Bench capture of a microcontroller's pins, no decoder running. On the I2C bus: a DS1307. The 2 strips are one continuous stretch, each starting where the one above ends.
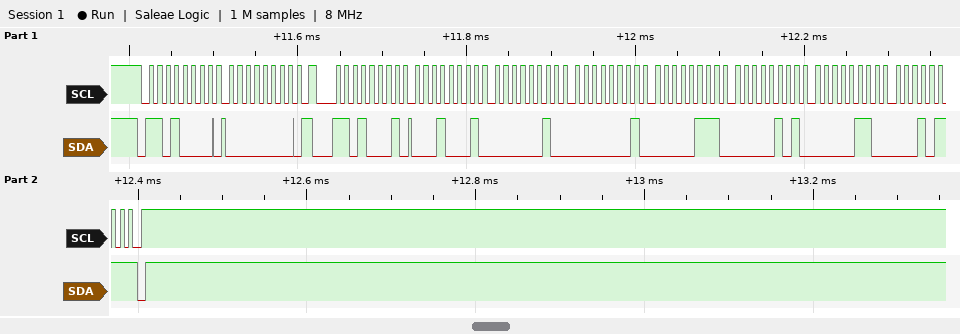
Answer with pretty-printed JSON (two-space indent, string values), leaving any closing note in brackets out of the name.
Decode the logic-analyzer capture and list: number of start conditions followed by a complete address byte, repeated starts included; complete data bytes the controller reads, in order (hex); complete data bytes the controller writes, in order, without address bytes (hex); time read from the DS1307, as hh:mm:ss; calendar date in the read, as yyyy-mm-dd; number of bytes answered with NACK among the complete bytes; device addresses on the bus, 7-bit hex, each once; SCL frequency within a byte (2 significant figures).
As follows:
{
  "number of start conditions followed by a complete address byte, repeated starts included": "2",
  "complete data bytes the controller reads, in order": "11 02 01 07 05 06 17",
  "complete data bytes the controller writes, in order, without address bytes": "00",
  "time read from the DS1307, as hh:mm:ss": "01:02:11",
  "calendar date in the read, as yyyy-mm-dd": "2017-06-05",
  "number of bytes answered with NACK among the complete bytes": "1",
  "device addresses on the bus, 7-bit hex, each once": "0x68",
  "SCL frequency within a byte": "100 kHz"
}
